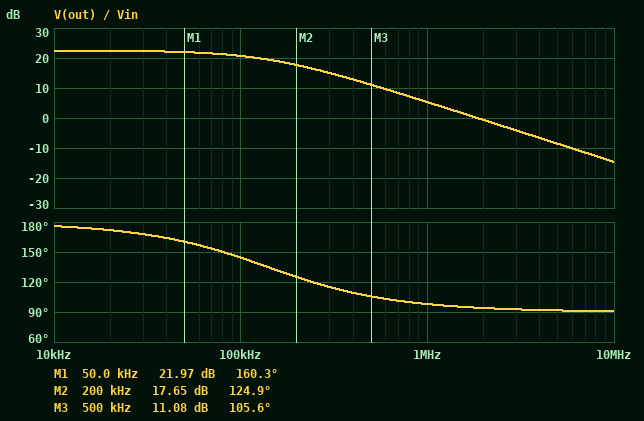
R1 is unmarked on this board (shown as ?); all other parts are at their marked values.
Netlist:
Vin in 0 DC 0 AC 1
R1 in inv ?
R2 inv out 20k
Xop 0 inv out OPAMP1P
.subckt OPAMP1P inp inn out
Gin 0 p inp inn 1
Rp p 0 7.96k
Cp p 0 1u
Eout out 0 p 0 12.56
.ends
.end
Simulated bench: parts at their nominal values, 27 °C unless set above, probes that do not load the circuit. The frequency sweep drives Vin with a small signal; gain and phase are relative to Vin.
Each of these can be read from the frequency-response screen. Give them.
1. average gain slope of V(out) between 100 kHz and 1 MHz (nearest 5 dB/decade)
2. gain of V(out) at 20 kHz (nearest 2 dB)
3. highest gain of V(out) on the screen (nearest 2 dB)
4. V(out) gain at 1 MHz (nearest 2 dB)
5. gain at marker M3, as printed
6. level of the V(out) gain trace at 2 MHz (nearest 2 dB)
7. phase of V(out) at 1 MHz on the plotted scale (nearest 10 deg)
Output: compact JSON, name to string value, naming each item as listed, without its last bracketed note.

{"average gain slope of V(out) between 100 kHz and 1 MHz": "-15 dB/decade", "gain of V(out) at 20 kHz": "22 dB", "highest gain of V(out) on the screen": "22 dB", "V(out) gain at 1 MHz": "6 dB", "gain at marker M3, as printed": "11.08 dB", "level of the V(out) gain trace at 2 MHz": "0 dB", "phase of V(out) at 1 MHz on the plotted scale": "100 deg"}
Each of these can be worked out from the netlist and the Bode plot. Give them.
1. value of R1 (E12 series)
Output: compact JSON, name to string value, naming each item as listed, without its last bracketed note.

{"value of R1": "1.5 kΩ"}
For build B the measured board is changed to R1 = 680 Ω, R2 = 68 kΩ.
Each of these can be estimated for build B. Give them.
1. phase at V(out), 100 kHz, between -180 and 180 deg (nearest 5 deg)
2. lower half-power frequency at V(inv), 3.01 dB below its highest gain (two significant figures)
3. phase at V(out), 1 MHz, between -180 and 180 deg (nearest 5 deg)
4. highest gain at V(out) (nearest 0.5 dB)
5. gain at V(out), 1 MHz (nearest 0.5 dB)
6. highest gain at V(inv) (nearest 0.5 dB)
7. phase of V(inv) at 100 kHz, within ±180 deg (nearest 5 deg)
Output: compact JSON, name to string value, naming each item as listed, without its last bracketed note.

{"phase at V(out), 100 kHz, between -180 and 180 deg": "100 deg", "lower half-power frequency at V(inv), 3.01 dB below its highest gain": "20 kHz", "phase at V(out), 1 MHz, between -180 and 180 deg": "90 deg", "highest gain at V(out)": "40.0 dB", "gain at V(out), 1 MHz": "6.0 dB", "highest gain at V(inv)": "0 dB", "phase of V(inv) at 100 kHz, within ±180 deg": "10 deg"}
